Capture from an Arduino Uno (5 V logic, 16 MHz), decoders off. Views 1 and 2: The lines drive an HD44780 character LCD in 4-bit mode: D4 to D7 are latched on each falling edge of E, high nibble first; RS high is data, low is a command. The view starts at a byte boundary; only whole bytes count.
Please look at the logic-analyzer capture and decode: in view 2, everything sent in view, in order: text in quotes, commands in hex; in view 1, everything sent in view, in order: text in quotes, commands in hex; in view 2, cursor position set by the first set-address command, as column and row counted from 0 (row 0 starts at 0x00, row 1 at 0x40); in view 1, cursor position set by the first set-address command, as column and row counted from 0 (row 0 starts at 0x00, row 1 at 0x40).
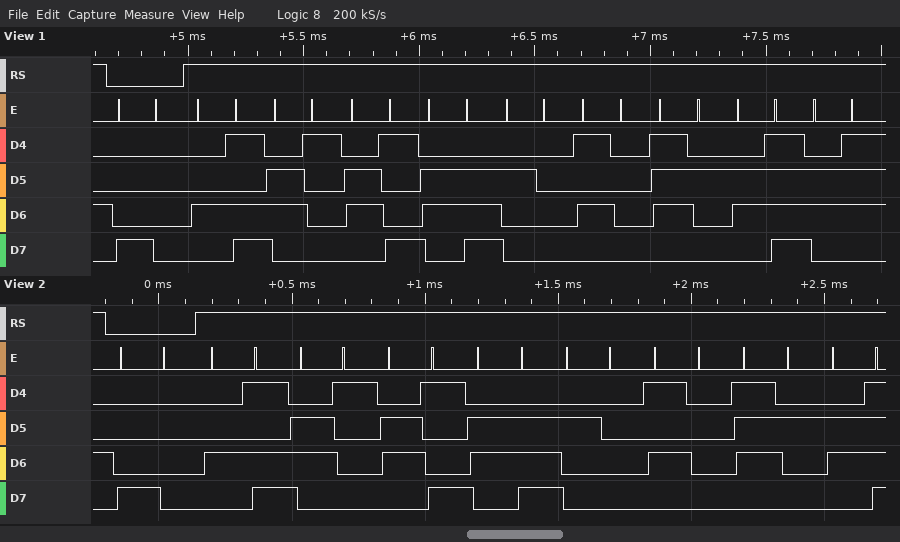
0x80 "Main Pro"
0x80 "Main Prog"
column 0, row 0
column 0, row 0
